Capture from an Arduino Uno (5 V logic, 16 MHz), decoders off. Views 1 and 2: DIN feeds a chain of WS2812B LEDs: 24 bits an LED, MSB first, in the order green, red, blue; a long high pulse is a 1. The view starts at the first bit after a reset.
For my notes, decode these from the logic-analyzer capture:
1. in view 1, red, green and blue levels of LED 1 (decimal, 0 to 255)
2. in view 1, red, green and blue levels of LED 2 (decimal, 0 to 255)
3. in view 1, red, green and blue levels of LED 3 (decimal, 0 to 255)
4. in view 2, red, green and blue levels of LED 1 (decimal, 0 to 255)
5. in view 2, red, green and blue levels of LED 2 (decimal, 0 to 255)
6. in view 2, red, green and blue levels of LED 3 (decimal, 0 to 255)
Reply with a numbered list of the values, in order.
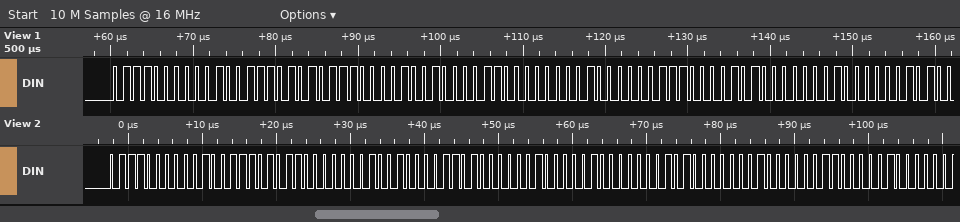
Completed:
1. 39, 112, 87
2. 12, 9, 2
3. 10, 7, 2
4. 39, 112, 88
5. 13, 9, 2
6. 10, 8, 2
